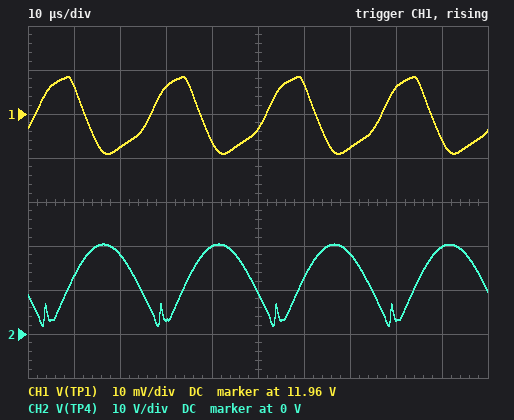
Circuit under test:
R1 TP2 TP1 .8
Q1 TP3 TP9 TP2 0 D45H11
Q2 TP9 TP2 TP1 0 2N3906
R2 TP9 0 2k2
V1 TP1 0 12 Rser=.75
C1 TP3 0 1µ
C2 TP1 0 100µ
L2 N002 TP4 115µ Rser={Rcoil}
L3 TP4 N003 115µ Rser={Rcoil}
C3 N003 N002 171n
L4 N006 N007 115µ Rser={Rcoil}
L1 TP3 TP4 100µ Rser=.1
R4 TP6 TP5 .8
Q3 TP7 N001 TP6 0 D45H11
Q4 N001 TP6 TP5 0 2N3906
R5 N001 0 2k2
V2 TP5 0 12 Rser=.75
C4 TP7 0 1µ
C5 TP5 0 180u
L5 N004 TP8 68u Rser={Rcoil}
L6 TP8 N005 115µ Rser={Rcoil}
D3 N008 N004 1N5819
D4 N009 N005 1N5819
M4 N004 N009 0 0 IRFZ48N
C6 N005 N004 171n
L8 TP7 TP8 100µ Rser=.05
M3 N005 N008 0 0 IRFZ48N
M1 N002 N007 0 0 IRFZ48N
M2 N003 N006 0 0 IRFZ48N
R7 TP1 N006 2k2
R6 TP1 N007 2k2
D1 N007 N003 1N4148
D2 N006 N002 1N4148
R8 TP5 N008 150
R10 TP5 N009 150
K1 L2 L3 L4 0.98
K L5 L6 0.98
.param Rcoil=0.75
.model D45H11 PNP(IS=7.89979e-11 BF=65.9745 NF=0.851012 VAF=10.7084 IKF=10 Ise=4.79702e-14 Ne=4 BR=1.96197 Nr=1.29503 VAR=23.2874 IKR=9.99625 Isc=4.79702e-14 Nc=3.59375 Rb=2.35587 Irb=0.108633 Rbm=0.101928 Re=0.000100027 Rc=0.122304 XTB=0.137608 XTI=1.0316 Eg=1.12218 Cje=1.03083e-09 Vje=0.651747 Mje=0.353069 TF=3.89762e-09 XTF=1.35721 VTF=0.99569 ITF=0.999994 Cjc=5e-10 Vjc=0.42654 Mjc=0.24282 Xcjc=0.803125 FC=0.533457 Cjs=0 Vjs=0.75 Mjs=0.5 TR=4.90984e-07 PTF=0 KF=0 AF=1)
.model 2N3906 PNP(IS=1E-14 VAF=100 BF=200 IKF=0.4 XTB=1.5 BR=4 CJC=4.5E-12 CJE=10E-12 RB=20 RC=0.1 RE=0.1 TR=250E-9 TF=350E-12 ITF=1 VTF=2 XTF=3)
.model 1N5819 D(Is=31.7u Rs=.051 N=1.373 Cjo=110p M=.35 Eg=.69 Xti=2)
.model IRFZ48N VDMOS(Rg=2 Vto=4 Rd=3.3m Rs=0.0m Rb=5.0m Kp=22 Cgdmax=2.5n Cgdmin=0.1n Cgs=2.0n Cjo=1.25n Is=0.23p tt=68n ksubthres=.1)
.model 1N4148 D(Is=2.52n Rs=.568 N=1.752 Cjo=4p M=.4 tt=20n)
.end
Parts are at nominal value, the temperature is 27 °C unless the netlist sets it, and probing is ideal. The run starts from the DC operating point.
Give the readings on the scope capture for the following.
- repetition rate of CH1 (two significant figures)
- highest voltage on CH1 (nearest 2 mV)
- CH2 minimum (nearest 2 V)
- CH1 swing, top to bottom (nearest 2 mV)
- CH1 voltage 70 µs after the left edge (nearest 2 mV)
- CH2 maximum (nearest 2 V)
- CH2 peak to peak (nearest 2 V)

40 kHz
11.968 V
2 V
18 mV
11.952 V
20 V
18 V
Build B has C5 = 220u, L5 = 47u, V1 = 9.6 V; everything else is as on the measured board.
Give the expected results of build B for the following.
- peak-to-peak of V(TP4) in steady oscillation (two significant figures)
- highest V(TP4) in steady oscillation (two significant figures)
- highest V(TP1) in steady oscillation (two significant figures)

15 V
16 V
9.6 V
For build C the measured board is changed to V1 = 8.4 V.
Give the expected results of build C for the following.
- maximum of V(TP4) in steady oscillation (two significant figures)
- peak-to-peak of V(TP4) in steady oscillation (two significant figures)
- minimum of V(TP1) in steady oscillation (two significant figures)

14 V
13 V
8.4 V
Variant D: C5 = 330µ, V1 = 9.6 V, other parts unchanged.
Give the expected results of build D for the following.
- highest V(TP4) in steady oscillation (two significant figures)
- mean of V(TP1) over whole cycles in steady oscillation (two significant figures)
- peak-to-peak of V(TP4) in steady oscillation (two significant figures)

16 V
9.6 V
15 V
